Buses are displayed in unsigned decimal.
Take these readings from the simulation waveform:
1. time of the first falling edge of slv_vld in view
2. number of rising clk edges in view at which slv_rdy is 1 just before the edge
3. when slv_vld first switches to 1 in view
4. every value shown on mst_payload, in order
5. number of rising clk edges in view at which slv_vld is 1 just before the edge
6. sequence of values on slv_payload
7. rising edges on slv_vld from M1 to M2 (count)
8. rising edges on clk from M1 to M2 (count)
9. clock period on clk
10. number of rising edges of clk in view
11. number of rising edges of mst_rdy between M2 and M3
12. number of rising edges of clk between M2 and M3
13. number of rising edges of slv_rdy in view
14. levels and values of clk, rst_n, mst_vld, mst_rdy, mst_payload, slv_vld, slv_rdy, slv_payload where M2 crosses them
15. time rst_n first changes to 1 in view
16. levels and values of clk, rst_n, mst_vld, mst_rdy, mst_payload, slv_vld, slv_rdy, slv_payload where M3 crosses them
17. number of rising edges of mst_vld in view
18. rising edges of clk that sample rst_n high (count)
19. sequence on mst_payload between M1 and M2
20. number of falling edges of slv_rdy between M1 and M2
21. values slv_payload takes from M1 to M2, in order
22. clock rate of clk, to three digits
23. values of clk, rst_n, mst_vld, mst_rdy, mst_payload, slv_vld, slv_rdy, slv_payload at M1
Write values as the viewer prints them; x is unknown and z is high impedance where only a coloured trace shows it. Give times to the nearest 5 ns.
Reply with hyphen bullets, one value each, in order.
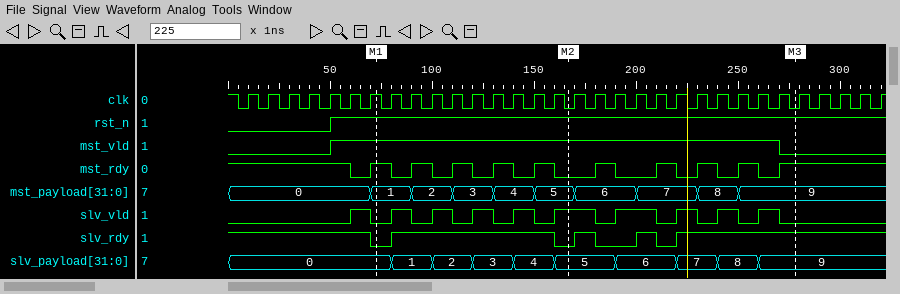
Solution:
- 70 ns
- 27
- 60 ns
- 0, 1, 2, 3, 4, 5, 6, 7, 8, 9
- 12
- 0, 1, 2, 3, 4, 5, 6, 7, 8, 9
- 5
- 9
- 10 ns
- 32
- 5
- 11
- 4
- clk=0, rst_n=1, mst_vld=1, mst_rdy=0, mst_payload=5, slv_vld=1, slv_rdy=0, slv_payload=5
- 50 ns
- clk=0, rst_n=1, mst_vld=0, mst_rdy=1, mst_payload=9, slv_vld=0, slv_rdy=1, slv_payload=9
- 1
- 27
- 1, 2, 3, 4, 5
- 1
- 0, 1, 2, 3, 4, 5
- 100 MHz
- clk=1, rst_n=1, mst_vld=1, mst_rdy=1, mst_payload=1, slv_vld=0, slv_rdy=0, slv_payload=0
